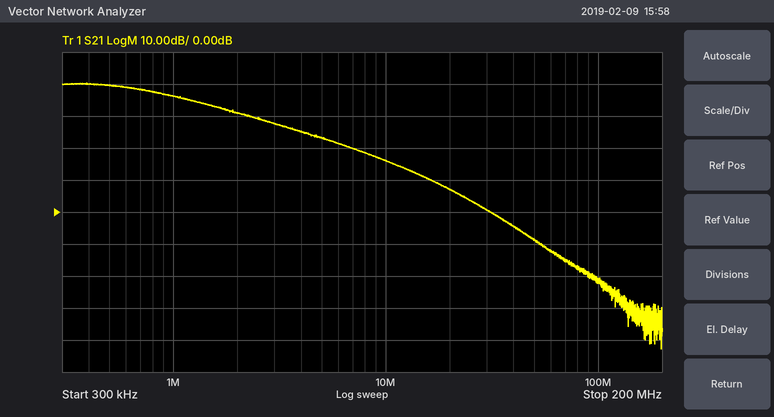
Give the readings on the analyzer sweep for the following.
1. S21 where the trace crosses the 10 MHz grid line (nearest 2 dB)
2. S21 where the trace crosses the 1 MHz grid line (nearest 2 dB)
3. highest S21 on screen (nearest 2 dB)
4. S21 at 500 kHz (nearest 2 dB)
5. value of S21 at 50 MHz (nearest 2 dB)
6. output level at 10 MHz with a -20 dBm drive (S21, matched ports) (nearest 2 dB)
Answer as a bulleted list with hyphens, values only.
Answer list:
- 16 dB
- 36 dB
- 40 dB
- 40 dB
- -8 dB
- -4 dBm
